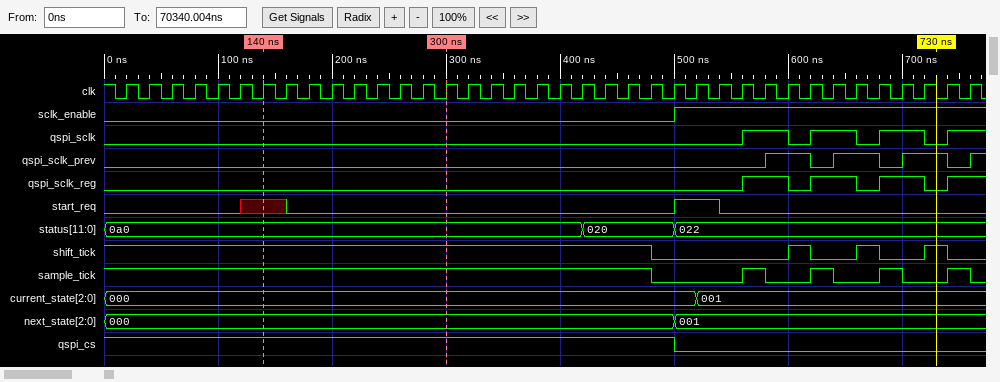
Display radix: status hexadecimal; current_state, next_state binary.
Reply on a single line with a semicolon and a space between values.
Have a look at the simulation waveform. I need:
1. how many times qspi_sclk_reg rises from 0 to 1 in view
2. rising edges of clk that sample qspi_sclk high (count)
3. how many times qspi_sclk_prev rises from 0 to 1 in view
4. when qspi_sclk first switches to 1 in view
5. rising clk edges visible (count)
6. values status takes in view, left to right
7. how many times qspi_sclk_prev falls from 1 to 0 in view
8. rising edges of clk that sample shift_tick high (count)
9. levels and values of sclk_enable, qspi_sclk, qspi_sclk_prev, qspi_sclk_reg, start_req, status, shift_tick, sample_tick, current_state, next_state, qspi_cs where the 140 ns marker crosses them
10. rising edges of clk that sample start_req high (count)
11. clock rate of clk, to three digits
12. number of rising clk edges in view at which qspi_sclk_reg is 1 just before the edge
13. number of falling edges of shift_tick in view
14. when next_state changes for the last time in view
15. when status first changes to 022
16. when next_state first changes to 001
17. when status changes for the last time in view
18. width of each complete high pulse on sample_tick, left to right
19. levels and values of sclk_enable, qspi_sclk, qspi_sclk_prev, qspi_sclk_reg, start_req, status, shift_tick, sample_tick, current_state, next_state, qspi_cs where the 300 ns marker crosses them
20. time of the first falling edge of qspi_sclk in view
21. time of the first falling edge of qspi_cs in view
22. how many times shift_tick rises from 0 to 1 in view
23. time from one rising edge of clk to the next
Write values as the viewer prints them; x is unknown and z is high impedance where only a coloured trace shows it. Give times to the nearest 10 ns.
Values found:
4; 7; 4; 560 ns; 38; 0a0, 020, 022; 3; 27; sclk_enable=0, qspi_sclk=0, qspi_sclk_prev=0, qspi_sclk_reg=0, start_req=x, status=0a0, shift_tick=1, sample_tick=1, current_state=000, next_state=000, qspi_cs=1; 2; 50.0 MHz; 7; 4; 500 ns; 500 ns; 500 ns; 500 ns; 20 ns, 20 ns, 20 ns, 20 ns; sclk_enable=0, qspi_sclk=0, qspi_sclk_prev=0, qspi_sclk_reg=0, start_req=0, status=0a0, shift_tick=1, sample_tick=1, current_state=000, next_state=000, qspi_cs=1; 600 ns; 500 ns; 3; 20 ns
